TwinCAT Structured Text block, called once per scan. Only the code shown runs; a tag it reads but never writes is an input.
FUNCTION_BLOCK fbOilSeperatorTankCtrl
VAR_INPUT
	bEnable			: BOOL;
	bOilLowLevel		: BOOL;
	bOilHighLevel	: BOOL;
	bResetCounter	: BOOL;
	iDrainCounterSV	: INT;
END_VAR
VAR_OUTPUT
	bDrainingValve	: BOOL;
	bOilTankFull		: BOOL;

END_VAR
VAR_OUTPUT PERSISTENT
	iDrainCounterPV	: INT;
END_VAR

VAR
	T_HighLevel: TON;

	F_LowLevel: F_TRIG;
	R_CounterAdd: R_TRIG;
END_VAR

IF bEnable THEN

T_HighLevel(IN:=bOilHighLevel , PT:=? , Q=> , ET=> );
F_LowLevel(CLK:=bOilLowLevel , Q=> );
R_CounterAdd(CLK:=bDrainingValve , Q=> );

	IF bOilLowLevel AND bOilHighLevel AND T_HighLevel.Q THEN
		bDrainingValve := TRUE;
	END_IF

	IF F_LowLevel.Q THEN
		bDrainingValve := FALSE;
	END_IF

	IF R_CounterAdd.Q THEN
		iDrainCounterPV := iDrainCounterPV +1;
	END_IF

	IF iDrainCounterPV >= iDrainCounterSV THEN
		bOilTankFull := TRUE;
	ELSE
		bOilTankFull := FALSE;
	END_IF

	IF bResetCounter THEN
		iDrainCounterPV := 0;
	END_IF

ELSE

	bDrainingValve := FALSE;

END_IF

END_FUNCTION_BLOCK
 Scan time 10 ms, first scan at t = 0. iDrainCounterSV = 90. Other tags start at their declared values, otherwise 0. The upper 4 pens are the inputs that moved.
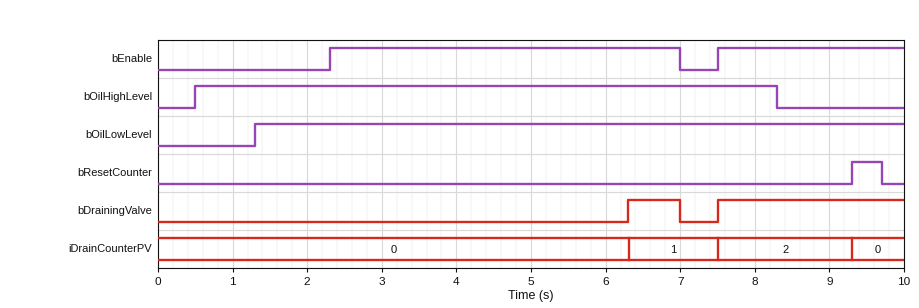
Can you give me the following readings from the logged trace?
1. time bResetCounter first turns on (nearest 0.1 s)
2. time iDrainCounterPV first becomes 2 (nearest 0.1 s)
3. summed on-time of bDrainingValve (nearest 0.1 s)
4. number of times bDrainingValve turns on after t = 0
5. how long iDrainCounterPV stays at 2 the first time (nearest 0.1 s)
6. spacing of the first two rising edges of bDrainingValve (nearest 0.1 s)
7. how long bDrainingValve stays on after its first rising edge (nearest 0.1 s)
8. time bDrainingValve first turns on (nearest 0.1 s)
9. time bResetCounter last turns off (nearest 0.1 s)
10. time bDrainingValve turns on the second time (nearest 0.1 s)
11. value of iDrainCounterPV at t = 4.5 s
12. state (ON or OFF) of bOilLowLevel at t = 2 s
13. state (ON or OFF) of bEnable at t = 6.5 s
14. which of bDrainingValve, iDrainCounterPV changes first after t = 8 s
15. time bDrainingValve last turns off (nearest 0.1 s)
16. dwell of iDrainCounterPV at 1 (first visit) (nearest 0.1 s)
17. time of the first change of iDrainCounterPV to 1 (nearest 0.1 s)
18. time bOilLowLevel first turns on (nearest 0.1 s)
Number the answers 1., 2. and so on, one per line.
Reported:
1. 9.3 s
2. 7.5 s
3. 3.2 s
4. 2
5. 1.8 s
6. 1.2 s
7. 0.7 s
8. 6.3 s
9. 9.7 s
10. 7.5 s
11. 0
12. ON
13. ON
14. iDrainCounterPV
15. 7.0 s
16. 1.2 s
17. 6.3 s
18. 1.3 s
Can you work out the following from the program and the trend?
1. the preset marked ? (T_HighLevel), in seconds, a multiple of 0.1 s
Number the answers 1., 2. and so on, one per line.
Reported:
1. 4.0 s
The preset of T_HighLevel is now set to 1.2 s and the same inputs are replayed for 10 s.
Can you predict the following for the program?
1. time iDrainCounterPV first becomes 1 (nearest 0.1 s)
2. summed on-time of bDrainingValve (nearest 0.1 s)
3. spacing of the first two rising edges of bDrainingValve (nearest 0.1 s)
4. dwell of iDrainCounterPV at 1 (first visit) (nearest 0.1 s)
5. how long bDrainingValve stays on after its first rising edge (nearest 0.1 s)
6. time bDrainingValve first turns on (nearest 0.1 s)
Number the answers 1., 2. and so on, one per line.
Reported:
1. 3.5 s
2. 6.0 s
3. 4.0 s
4. 4.0 s
5. 3.5 s
6. 3.5 s
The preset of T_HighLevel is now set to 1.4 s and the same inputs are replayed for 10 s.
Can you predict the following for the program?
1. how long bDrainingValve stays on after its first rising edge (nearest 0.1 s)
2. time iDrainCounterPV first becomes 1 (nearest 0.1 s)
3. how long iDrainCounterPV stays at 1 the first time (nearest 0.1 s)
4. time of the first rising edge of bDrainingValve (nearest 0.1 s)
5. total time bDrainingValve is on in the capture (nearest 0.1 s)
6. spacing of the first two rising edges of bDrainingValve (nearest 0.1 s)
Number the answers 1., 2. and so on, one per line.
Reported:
1. 3.3 s
2. 3.7 s
3. 3.8 s
4. 3.7 s
5. 5.8 s
6. 3.8 s
